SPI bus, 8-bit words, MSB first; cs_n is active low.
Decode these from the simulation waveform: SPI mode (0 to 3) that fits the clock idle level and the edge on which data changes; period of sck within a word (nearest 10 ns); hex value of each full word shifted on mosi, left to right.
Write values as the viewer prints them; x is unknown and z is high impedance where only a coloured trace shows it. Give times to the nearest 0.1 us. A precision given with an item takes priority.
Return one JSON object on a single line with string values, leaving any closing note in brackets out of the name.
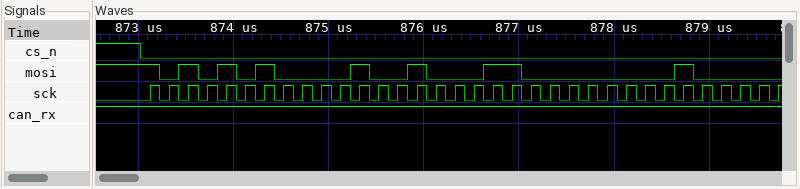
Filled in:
{"SPI mode (0 to 3) that fits the clock idle level and the edge on which data changes": "0", "period of sck within a word": "200 ns", "hex value of each full word shifted on mosi, left to right": "AA, 12, 30, 08"}
